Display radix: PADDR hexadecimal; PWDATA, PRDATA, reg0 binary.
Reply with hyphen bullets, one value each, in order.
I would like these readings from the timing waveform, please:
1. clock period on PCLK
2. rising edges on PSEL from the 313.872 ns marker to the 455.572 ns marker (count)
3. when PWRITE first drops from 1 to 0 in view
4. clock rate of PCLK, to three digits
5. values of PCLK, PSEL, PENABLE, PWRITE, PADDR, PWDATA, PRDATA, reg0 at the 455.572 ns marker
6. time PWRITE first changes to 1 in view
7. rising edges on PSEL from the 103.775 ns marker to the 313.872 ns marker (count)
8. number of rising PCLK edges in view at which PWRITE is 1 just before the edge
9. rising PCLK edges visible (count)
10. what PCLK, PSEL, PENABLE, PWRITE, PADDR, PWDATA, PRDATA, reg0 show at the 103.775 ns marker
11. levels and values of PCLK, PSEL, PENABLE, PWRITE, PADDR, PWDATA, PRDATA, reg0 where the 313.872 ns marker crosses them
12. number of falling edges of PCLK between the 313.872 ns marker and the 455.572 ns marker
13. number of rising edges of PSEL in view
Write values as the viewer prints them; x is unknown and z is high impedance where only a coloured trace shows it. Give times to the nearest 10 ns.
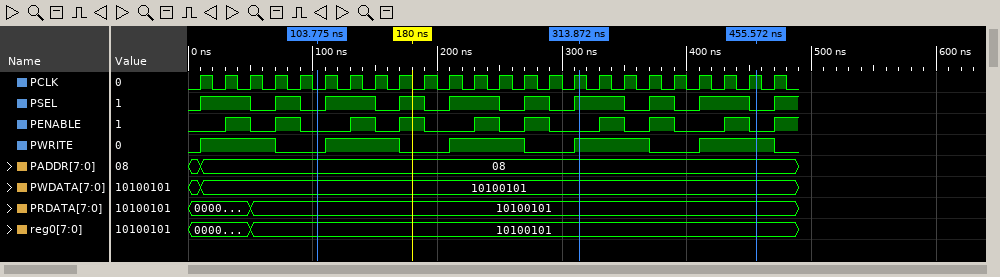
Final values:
- 20 ns
- 2
- 70 ns
- 50.0 MHz
- PCLK=1, PSEL=0, PENABLE=0, PWRITE=1, PADDR=08, PWDATA=10100101, PRDATA=10100101, reg0=10100101
- 10 ns
- 5
- 15
- 24
- PCLK=0, PSEL=0, PENABLE=0, PWRITE=0, PADDR=08, PWDATA=10100101, PRDATA=10100101, reg0=10100101
- PCLK=1, PSEL=1, PENABLE=0, PWRITE=1, PADDR=08, PWDATA=10100101, PRDATA=10100101, reg0=10100101
- 7
- 10
